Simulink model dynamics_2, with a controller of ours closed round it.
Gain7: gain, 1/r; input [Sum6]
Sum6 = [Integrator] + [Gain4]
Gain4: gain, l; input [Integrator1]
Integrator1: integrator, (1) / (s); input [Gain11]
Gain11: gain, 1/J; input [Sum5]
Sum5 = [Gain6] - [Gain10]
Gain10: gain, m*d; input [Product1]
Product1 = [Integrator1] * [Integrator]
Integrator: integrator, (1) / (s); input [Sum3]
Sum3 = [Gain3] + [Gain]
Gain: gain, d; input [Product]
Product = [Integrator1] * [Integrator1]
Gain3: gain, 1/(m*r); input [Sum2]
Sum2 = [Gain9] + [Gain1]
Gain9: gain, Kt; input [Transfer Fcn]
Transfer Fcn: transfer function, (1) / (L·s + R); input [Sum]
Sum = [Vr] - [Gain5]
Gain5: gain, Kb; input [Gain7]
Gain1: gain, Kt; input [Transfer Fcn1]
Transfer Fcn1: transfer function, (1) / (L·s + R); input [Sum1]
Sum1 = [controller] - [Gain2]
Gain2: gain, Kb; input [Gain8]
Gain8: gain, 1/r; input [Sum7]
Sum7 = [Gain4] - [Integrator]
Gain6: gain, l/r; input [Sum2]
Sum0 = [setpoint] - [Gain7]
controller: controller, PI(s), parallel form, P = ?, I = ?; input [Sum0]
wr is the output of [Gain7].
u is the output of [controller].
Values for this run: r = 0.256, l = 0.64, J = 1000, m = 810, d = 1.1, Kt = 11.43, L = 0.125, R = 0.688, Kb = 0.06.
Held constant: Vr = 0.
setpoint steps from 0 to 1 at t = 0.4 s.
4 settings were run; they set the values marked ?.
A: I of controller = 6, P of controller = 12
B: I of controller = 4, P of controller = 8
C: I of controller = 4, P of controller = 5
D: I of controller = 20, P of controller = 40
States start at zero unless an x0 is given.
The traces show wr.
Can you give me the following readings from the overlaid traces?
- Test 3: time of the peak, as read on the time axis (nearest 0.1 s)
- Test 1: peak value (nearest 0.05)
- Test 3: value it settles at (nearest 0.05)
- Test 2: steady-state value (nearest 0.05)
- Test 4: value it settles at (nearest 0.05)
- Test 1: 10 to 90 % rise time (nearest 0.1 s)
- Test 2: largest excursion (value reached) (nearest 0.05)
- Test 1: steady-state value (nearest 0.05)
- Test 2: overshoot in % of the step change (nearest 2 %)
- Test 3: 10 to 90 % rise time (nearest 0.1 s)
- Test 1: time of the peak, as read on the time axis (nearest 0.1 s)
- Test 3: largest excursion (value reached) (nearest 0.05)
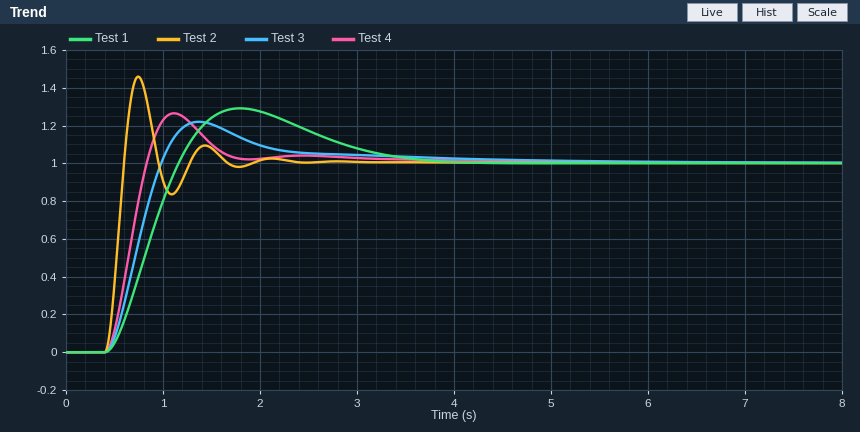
1.4 s
1.30
1.00
1.00
1.00
0.5 s
1.45
1.00
46 %
0.4 s
1.8 s
1.20
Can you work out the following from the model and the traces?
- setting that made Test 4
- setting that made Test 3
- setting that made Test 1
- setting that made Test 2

A
B
C
D
